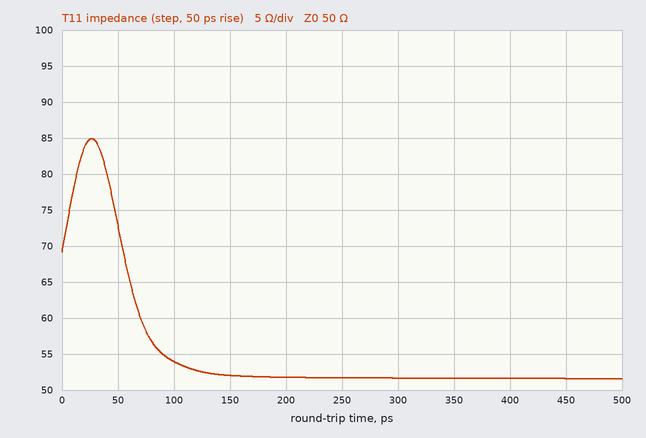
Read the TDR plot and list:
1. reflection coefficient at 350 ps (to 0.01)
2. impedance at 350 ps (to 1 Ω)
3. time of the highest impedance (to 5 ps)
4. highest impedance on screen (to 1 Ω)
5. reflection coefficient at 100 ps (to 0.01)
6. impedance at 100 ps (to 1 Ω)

+0.02
52 Ω
25 ps
85 Ω
+0.04
54 Ω
